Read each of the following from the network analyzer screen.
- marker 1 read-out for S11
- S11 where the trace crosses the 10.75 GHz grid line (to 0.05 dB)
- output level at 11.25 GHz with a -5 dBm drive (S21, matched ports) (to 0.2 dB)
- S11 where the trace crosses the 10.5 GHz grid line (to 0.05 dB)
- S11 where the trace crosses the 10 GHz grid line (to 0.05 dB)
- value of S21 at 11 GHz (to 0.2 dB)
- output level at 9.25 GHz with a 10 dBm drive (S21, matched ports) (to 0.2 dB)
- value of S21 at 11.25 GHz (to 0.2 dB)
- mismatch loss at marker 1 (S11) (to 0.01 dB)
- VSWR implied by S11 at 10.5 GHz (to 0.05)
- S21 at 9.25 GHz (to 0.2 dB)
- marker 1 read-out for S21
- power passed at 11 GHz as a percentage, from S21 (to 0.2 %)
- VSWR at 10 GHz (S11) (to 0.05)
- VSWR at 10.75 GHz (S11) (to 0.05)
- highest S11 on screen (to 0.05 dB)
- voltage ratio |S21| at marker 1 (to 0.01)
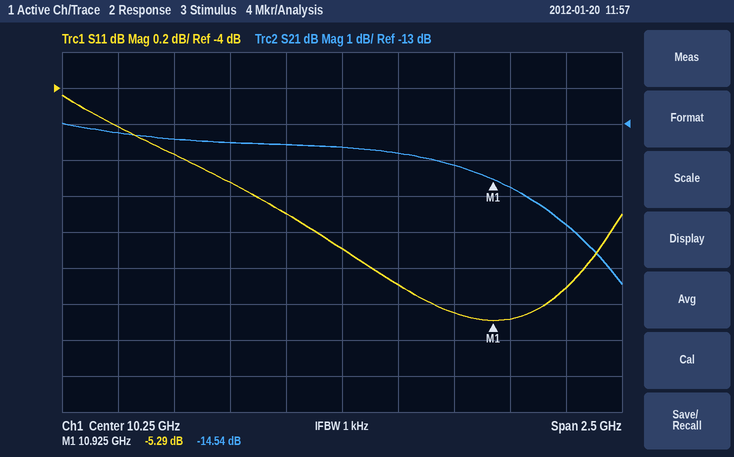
-5.29 dB
-5.25 dB
-20.8 dBm
-5.10 dB
-4.70 dB
-14.8 dB
-3.2 dBm
-15.8 dB
1.52 dB
3.50
-13.2 dB
-14.54 dB
3.4 %
3.80
3.40
-4.05 dB
0.19
